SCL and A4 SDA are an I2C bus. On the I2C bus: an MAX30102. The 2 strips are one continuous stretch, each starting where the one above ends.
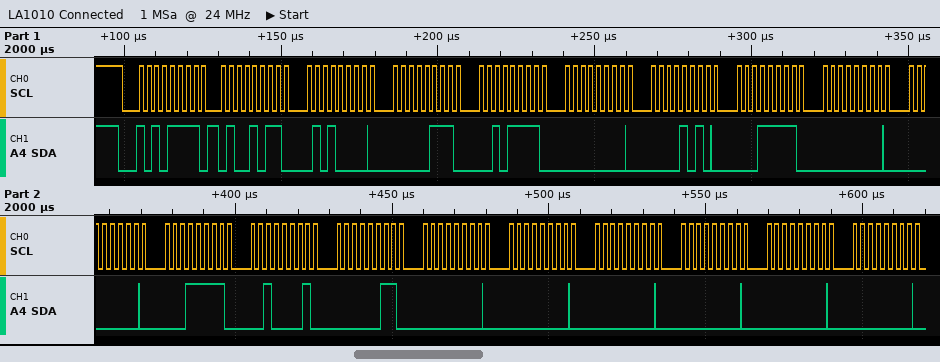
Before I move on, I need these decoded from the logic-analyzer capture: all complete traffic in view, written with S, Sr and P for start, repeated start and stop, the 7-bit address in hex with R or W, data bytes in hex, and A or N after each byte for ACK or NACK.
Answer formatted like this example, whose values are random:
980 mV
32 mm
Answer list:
S 57R A 4B A 50 A 07 A 2F A 00 A 0A A 1F A 00 A 00 A 1F A 21 A 03 A 00 A 00 A 00 A 00 A 00 A 00 A
